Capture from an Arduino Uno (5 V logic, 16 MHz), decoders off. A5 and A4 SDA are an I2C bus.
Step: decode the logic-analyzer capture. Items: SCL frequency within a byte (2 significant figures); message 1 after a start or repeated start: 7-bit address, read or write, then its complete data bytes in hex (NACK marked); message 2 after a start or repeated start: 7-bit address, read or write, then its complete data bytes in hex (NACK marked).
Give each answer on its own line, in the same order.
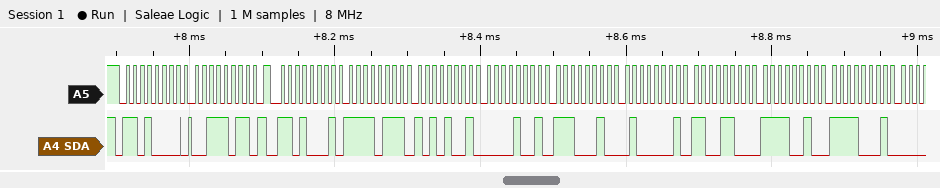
100 kHz
0x68 write: 3B
0x68 read: F7 A9 09 E2 41 CC F2 F1
